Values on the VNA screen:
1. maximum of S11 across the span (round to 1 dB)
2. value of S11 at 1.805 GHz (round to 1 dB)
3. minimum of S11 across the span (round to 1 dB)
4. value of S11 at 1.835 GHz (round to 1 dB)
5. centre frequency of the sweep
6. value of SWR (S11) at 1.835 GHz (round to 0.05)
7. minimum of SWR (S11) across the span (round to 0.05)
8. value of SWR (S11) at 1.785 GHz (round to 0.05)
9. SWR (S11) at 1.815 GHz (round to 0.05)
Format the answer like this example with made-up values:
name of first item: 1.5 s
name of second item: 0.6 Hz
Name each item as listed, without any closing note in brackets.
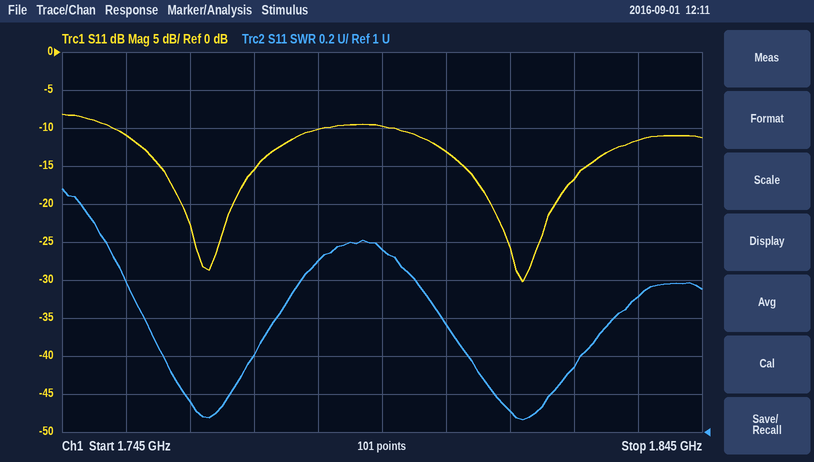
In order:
maximum of S11 across the span: -8 dB
value of S11 at 1.805 GHz: -13 dB
minimum of S11 across the span: -30 dB
value of S11 at 1.835 GHz: -12 dB
centre frequency of the sweep: 1.795 GHz
value of SWR (S11) at 1.835 GHz: 1.70
minimum of SWR (S11) across the span: 1.05
value of SWR (S11) at 1.785 GHz: 1.90
SWR (S11) at 1.815 GHz: 1.10
